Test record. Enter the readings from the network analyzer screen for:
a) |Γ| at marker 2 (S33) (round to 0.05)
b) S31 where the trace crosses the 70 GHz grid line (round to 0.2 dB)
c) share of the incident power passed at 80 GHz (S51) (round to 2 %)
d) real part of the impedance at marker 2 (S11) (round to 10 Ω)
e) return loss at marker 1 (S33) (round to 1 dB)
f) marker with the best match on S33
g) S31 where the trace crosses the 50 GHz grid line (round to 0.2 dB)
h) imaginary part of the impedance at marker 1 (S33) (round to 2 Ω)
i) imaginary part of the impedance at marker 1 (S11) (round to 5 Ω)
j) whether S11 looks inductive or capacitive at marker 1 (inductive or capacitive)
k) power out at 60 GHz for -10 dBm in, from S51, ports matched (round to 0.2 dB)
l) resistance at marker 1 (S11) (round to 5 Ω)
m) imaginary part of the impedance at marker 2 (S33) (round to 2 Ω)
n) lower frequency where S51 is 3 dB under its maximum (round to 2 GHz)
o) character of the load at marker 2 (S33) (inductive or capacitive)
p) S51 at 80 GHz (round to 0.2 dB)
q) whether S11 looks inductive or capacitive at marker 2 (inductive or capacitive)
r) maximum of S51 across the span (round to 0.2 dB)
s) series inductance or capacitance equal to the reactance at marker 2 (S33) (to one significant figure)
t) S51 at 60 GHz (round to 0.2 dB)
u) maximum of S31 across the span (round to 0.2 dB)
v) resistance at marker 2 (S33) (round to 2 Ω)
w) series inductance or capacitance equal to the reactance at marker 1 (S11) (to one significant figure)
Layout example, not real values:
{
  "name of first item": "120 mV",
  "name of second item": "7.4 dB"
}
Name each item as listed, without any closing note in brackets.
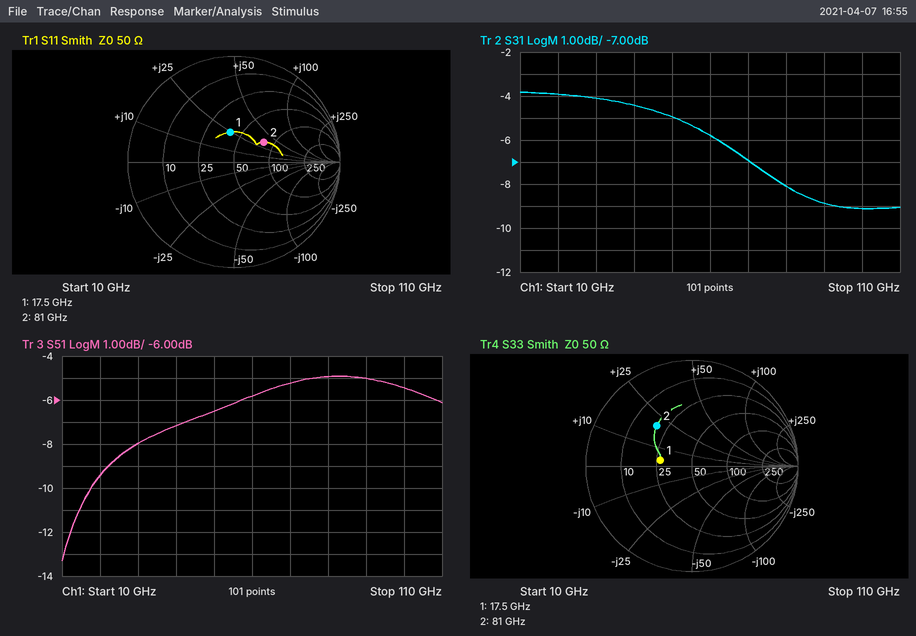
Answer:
{
  "|Γ| at marker 2 (S33)": "0.50",
  "S31 where the trace crosses the 70 GHz grid line": "-7.0 dB",
  "share of the incident power passed at 80 GHz (S51)": "32 %",
  "real part of the impedance at marker 2 (S11)": "80 Ω",
  "return loss at marker 1 (S33)": "10 dB",
  "marker with the best match on S33": "marker 1",
  "S31 where the trace crosses the 50 GHz grid line": "-5.0 dB",
  "imaginary part of the impedance at marker 1 (S33)": "+4 Ω",
  "imaginary part of the impedance at marker 1 (S11)": "+25 Ω",
  "whether S11 looks inductive or capacitive at marker 1": "inductive",
  "power out at 60 GHz for -10 dBm in, from S51, ports matched": "-15.8 dBm",
  "resistance at marker 1 (S11)": "40 Ω",
  "imaginary part of the impedance at marker 2 (S33)": "+20 Ω",
  "lower frequency where S51 is 3 dB under its maximum": "30 GHz",
  "character of the load at marker 2 (S33)": "inductive",
  "S51 at 80 GHz": "-5.0 dB",
  "whether S11 looks inductive or capacitive at marker 2": "inductive",
  "maximum of S51 across the span": "-5.0 dB",
  "series inductance or capacitance equal to the reactance at marker 2 (S33)": "40 pH",
  "S51 at 60 GHz": "-5.8 dB",
  "maximum of S31 across the span": "-3.8 dB",
  "resistance at marker 2 (S33)": "20 Ω",
  "series inductance or capacitance equal to the reactance at marker 1 (S11)": "200 pH"
}
